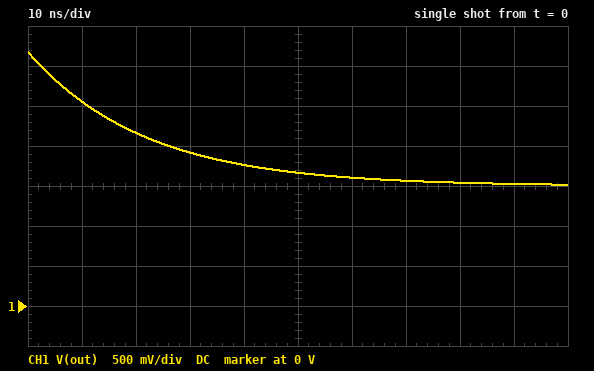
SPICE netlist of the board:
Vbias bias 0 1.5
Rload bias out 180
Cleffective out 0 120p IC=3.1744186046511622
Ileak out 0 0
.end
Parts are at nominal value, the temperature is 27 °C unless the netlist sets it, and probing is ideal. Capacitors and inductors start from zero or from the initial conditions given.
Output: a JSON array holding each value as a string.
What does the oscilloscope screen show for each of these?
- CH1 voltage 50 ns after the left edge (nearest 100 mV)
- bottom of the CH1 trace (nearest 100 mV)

["1.7 V", "1.5 V"]
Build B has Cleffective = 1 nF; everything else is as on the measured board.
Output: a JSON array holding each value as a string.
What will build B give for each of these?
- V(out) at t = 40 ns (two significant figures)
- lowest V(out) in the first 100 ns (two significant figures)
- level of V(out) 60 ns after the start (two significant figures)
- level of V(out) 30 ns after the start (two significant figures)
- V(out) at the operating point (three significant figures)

["2.8 V", "2.5 V", "2.7 V", "2.9 V", "1.50 V"]
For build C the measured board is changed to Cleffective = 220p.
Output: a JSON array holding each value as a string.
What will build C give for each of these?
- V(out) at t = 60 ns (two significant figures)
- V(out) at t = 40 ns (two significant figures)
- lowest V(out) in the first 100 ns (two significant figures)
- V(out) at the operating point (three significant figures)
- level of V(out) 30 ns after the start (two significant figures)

["1.9 V", "2.1 V", "1.6 V", "1.50 V", "2.3 V"]
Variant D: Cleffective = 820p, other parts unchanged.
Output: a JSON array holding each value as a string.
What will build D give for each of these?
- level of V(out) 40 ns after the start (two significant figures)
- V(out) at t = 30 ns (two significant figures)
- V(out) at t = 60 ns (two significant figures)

["2.8 V", "2.9 V", "2.6 V"]
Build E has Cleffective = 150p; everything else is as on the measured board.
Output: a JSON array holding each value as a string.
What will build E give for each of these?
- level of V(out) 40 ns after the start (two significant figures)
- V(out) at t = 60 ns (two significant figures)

["1.9 V", "1.7 V"]
